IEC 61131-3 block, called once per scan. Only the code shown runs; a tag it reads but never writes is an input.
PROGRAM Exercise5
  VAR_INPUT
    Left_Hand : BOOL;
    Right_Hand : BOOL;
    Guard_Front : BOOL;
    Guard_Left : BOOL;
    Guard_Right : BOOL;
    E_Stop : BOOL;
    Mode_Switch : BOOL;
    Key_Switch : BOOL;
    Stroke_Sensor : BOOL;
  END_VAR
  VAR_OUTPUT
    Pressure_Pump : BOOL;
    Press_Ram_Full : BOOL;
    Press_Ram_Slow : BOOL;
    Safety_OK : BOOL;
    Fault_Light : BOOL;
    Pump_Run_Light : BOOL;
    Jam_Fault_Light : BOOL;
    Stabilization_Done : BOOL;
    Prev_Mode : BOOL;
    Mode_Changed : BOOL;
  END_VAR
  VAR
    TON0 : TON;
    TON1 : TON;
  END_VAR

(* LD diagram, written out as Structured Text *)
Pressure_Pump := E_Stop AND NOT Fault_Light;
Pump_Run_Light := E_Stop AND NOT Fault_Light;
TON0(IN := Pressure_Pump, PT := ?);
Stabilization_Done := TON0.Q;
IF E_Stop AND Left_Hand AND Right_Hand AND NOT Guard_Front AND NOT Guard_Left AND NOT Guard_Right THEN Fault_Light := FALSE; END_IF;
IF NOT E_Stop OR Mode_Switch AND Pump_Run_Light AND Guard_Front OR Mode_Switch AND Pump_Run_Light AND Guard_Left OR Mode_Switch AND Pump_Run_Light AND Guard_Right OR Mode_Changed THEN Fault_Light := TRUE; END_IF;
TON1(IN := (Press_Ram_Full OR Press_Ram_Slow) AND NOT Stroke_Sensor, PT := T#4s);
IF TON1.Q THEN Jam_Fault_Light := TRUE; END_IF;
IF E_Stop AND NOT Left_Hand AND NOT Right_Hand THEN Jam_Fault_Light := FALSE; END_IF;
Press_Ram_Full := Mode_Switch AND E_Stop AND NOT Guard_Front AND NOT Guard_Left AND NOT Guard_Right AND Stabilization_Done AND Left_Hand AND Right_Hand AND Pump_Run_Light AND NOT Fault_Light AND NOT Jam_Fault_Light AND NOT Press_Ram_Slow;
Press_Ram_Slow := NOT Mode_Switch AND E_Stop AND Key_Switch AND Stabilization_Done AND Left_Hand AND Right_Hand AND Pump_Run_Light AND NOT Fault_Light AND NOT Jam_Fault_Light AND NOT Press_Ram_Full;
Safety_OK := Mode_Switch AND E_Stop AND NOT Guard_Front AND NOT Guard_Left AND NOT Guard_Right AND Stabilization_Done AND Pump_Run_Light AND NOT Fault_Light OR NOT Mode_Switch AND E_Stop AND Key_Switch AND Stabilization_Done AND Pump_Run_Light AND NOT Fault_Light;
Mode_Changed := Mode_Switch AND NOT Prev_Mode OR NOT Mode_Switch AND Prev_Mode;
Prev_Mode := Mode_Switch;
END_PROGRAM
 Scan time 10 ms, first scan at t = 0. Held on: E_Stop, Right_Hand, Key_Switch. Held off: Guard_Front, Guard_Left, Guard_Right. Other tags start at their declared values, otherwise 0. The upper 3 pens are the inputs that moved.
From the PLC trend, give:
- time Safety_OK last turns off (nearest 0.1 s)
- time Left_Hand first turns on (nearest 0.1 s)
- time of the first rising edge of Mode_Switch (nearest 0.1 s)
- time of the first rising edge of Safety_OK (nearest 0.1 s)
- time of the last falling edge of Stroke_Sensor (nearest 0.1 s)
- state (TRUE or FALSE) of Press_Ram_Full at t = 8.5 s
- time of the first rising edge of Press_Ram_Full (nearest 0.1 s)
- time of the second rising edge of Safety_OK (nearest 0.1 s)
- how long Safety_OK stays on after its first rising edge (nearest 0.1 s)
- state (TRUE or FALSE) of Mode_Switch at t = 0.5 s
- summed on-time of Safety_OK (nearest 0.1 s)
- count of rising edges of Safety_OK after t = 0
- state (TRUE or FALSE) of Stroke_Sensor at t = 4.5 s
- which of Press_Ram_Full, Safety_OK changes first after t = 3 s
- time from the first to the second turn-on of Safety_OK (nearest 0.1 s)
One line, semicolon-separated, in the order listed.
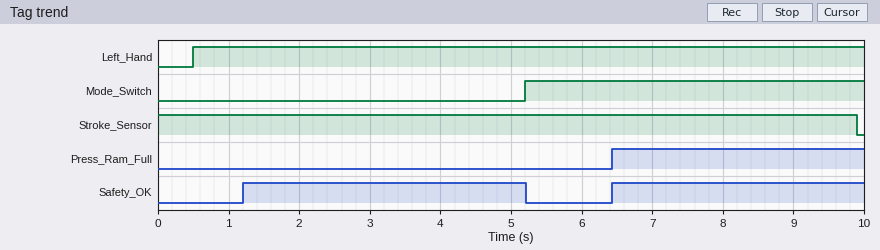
5.2 s; 0.5 s; 5.2 s; 1.2 s; 9.9 s; TRUE; 6.4 s; 6.4 s; 4.0 s; FALSE; 7.6 s; 2; TRUE; Safety_OK; 5.2 s
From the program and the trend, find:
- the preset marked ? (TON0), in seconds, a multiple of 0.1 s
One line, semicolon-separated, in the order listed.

1.2 s
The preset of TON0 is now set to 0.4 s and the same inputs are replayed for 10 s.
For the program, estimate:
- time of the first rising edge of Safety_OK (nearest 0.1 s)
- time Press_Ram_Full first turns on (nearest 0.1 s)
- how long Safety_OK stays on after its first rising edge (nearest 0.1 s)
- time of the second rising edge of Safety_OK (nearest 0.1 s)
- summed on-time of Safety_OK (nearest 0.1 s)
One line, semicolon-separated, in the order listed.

0.4 s; 5.6 s; 4.8 s; 5.6 s; 9.2 s
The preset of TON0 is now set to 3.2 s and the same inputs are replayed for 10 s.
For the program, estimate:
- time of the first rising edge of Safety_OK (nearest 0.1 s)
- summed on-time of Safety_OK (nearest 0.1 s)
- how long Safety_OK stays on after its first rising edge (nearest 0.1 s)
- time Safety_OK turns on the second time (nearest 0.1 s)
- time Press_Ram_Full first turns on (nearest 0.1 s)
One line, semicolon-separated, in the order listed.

3.2 s; 3.6 s; 2.0 s; 8.4 s; 8.4 s
